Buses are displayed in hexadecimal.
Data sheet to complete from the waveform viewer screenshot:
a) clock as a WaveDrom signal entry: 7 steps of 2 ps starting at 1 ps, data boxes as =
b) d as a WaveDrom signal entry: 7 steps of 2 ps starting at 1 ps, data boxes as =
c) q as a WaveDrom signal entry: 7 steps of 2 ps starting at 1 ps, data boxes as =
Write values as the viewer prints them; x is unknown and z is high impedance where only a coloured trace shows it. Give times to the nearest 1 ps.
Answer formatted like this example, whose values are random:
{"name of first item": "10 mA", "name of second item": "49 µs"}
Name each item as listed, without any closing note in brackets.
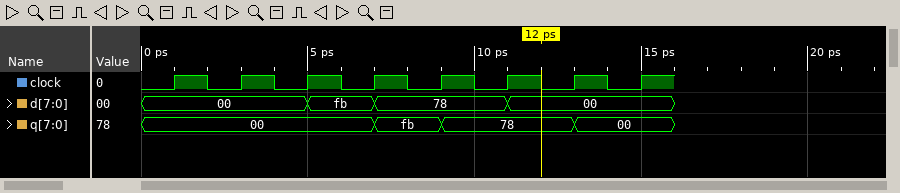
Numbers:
{"clock as a WaveDrom signal entry: 7 steps of 2 ps starting at 1 ps, data boxes as =": "{name: 'clock', wave: 'p......'}", "d as a WaveDrom signal entry: 7 steps of 2 ps starting at 1 ps, data boxes as =": "{name: 'd', wave: '=.==.=.', data: '00 fb 78 00'}", "q as a WaveDrom signal entry: 7 steps of 2 ps starting at 1 ps, data boxes as =": "{name: 'q', wave: '=..==.=', data: '00 fb 78 00'}"}
